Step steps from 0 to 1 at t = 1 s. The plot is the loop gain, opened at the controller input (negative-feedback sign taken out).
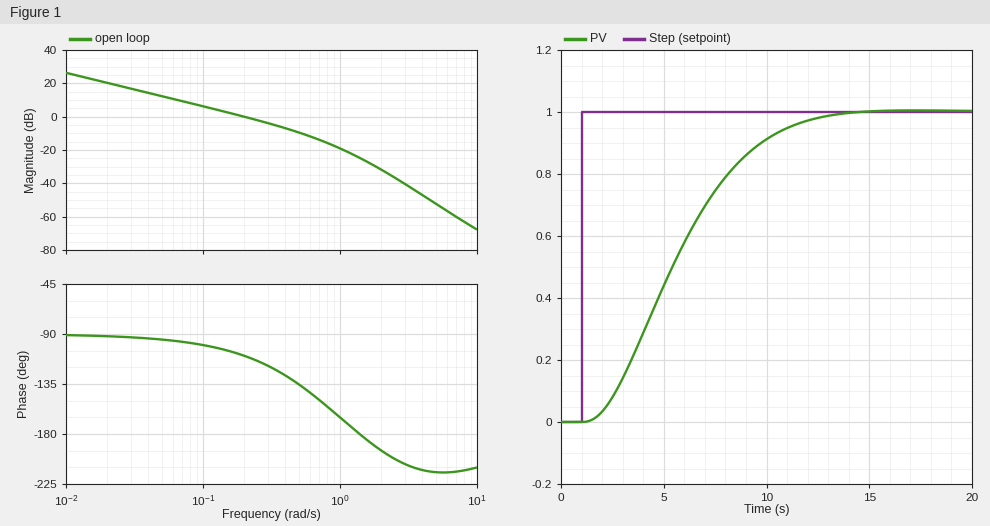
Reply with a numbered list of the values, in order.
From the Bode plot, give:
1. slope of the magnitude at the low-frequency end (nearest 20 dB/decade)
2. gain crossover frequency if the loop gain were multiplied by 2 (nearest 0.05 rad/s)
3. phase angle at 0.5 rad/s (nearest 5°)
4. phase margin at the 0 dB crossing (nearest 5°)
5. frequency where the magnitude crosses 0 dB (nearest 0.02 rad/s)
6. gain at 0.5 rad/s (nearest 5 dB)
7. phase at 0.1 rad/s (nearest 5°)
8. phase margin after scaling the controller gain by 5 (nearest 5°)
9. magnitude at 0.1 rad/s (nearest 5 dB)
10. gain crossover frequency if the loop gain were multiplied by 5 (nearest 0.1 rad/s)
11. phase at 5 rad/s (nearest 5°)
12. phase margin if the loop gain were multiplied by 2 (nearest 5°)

1. -20 dB/decade
2. 0.35 rad/s
3. -135°
4. 70°
5. 0.20 rad/s
6. -10 dB
7. -100°
8. 30°
9. 5 dB
10. 0.7 rad/s
11. -215°
12. 55°
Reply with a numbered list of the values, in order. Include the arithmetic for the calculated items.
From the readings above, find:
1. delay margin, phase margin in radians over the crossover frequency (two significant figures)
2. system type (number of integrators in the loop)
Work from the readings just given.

1. 70 × π / 180 / 0.2 = 6.1 s
2. 1
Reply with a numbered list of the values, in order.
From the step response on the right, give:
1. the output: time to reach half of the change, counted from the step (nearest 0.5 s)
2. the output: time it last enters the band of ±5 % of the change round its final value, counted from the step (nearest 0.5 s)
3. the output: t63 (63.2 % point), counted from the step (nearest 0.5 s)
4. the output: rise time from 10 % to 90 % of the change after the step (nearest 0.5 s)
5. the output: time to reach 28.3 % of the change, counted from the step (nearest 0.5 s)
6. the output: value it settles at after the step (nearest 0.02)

1. 4.5 s
2. 10.0 s
3. 5.5 s
4. 7.0 s
5. 3.0 s
6. 1.00
